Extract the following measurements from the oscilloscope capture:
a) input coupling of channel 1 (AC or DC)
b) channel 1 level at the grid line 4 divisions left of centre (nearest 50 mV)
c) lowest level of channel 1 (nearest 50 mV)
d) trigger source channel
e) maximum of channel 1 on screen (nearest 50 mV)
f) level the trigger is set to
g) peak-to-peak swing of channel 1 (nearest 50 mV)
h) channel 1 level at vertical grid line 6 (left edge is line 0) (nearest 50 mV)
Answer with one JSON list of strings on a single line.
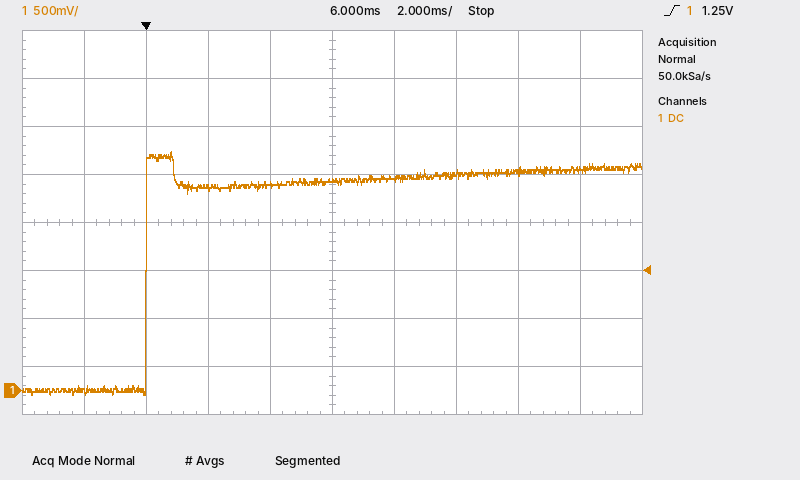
["DC", "0 mV", "-50 mV", "channel 1", "2.50 V", "1.25 V", "2.55 V", "2.20 V"]
